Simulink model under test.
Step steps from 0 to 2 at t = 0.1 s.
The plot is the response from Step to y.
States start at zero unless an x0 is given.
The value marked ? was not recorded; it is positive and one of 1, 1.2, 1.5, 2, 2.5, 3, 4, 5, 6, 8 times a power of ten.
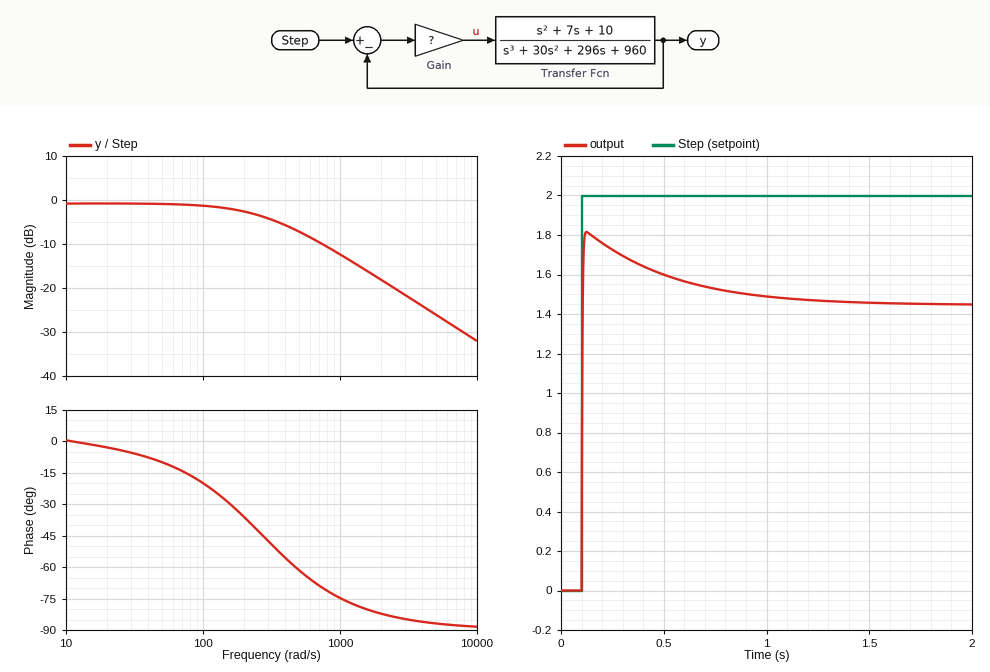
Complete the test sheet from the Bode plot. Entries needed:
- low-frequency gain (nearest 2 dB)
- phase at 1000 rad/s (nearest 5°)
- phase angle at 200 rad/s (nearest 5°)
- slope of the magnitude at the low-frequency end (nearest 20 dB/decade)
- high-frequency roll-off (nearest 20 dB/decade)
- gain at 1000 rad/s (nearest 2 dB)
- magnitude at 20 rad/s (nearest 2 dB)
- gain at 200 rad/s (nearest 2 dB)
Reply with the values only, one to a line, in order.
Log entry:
0 dB
-75°
-35°
0 dB/decade
-20 dB/decade
-12 dB
0 dB
-2 dB
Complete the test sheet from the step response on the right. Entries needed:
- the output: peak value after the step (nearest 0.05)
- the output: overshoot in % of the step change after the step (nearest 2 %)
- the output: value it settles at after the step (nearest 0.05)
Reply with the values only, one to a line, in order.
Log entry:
1.80
26 %
1.45
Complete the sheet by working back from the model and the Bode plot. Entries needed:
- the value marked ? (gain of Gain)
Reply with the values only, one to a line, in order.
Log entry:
250
